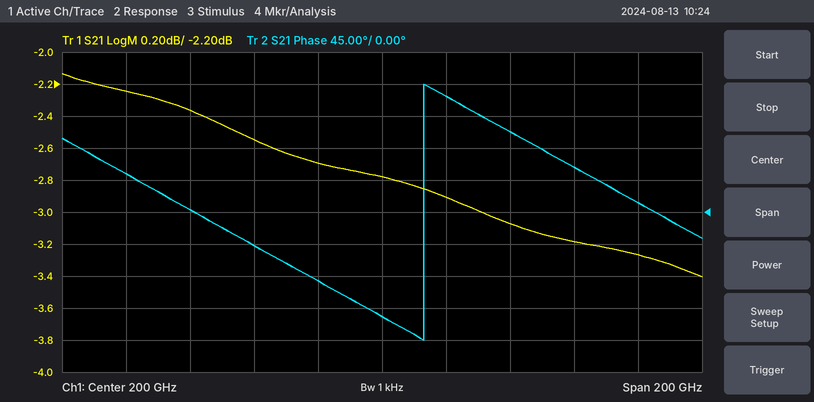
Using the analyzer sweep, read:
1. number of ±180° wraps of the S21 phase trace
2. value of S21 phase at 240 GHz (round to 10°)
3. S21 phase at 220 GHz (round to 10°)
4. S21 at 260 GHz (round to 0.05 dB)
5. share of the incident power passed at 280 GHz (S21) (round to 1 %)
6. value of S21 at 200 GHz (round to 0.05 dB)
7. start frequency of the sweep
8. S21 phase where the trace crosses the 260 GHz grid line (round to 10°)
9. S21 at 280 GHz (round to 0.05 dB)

1
110°
160°
-3.20 dB
47 %
-2.80 dB
100 GHz
60°
-3.25 dB
